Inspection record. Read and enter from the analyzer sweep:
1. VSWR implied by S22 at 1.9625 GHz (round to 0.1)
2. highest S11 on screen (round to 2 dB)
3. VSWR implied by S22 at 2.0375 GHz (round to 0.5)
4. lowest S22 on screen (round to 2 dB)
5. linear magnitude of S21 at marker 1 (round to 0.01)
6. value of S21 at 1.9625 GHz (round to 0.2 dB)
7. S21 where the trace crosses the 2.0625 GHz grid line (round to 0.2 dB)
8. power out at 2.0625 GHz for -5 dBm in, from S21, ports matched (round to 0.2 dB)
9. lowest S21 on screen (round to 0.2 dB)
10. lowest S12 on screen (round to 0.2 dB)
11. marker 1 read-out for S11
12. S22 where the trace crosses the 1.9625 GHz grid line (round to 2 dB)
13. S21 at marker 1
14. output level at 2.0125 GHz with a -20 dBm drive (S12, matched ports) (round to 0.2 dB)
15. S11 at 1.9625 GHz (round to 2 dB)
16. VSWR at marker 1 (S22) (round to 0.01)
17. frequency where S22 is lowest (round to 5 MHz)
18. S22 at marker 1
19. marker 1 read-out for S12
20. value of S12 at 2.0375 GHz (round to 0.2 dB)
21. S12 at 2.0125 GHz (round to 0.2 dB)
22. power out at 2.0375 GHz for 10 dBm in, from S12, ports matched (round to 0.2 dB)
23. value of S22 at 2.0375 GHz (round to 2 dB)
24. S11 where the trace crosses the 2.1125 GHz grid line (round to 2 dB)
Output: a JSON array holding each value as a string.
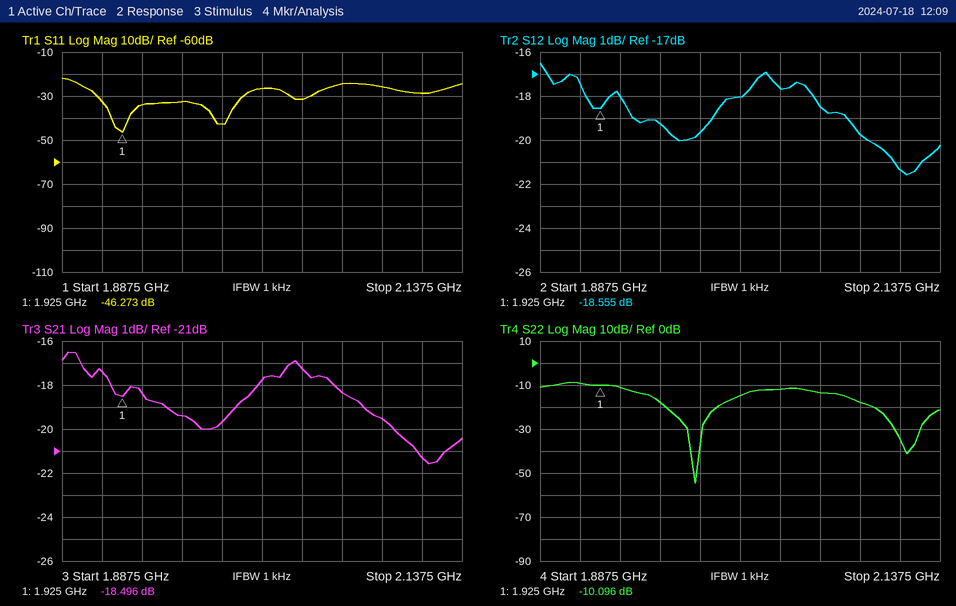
["1.3", "-22 dB", "1.5", "-54 dB", "0.12", "-19.4 dB", "-18.4 dB", "-23.4 dBm", "-21.6 dB", "-21.6 dB", "-46.273 dB", "-18 dB", "-18.496 dB", "-38.0 dBm", "-32 dB", "1.91", "1.985 GHz", "-10.096 dB", "-18.555 dB", "-17.6 dB", "-18.0 dB", "-7.6 dBm", "-12 dB", "-28 dB"]
